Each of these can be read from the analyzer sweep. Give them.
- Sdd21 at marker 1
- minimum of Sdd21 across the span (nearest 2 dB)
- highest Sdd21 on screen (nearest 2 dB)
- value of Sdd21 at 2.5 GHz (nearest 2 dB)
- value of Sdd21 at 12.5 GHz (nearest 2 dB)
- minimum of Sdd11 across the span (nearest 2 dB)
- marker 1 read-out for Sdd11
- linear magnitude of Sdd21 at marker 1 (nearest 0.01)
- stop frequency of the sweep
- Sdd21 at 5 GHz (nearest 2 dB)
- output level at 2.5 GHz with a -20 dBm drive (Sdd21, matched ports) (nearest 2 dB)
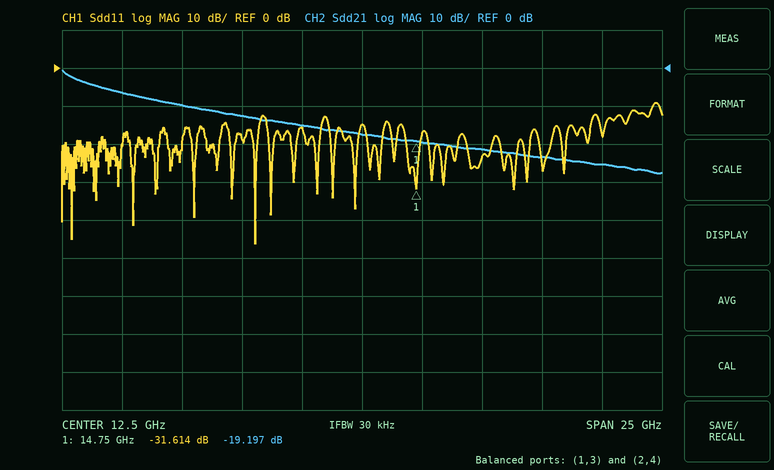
-19.197 dB
-28 dB
0 dB
-6 dB
-18 dB
-46 dB
-31.614 dB
0.11
25 GHz
-10 dB
-26 dBm
